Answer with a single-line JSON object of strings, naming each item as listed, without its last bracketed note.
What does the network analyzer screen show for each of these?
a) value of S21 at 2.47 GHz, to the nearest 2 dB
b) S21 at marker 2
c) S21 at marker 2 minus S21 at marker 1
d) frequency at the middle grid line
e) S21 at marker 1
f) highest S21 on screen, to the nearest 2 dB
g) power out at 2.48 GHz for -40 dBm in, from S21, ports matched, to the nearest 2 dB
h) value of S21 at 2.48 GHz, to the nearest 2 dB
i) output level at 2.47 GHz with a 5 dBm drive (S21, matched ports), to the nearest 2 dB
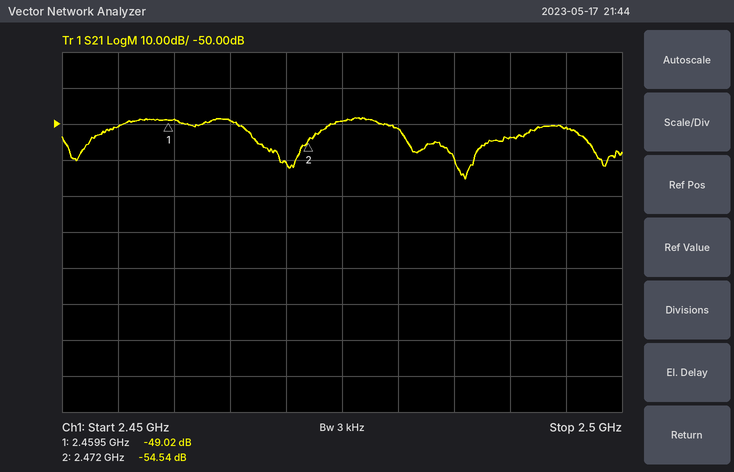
{"value of S21 at 2.47 GHz, to the nearest 2 dB": "-60 dB", "S21 at marker 2": "-54.54 dB", "S21 at marker 2 minus S21 at marker 1": "-5.52 dB", "frequency at the middle grid line": "2.475 GHz", "S21 at marker 1": "-49.02 dB", "highest S21 on screen, to the nearest 2 dB": "-48 dB", "power out at 2.48 GHz for -40 dBm in, from S21, ports matched, to the nearest 2 dB": "-92 dBm", "value of S21 at 2.48 GHz, to the nearest 2 dB": "-52 dB", "output level at 2.47 GHz with a 5 dBm drive (S21, matched ports), to the nearest 2 dB": "-56 dBm"}
